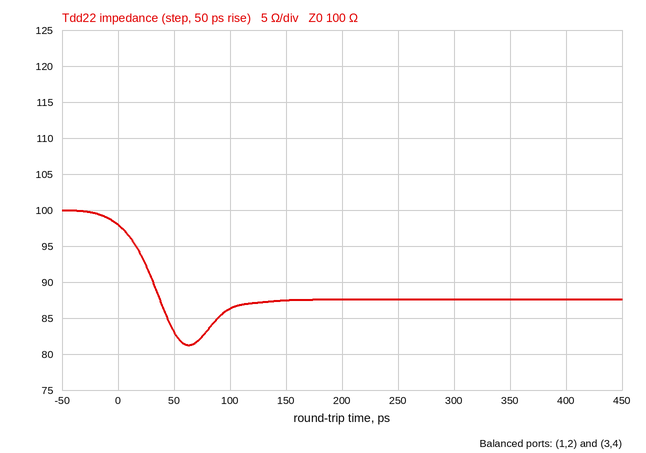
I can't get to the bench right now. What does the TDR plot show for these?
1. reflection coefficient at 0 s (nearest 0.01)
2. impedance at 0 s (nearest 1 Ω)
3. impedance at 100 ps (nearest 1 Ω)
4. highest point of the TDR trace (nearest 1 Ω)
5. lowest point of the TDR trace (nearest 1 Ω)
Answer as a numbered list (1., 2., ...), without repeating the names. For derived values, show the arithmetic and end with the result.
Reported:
1. (98 − 100)/(98 + 100) ≈ -0.01
2. 98 Ω
3. 86 Ω
4. 100 Ω
5. 81 Ω
